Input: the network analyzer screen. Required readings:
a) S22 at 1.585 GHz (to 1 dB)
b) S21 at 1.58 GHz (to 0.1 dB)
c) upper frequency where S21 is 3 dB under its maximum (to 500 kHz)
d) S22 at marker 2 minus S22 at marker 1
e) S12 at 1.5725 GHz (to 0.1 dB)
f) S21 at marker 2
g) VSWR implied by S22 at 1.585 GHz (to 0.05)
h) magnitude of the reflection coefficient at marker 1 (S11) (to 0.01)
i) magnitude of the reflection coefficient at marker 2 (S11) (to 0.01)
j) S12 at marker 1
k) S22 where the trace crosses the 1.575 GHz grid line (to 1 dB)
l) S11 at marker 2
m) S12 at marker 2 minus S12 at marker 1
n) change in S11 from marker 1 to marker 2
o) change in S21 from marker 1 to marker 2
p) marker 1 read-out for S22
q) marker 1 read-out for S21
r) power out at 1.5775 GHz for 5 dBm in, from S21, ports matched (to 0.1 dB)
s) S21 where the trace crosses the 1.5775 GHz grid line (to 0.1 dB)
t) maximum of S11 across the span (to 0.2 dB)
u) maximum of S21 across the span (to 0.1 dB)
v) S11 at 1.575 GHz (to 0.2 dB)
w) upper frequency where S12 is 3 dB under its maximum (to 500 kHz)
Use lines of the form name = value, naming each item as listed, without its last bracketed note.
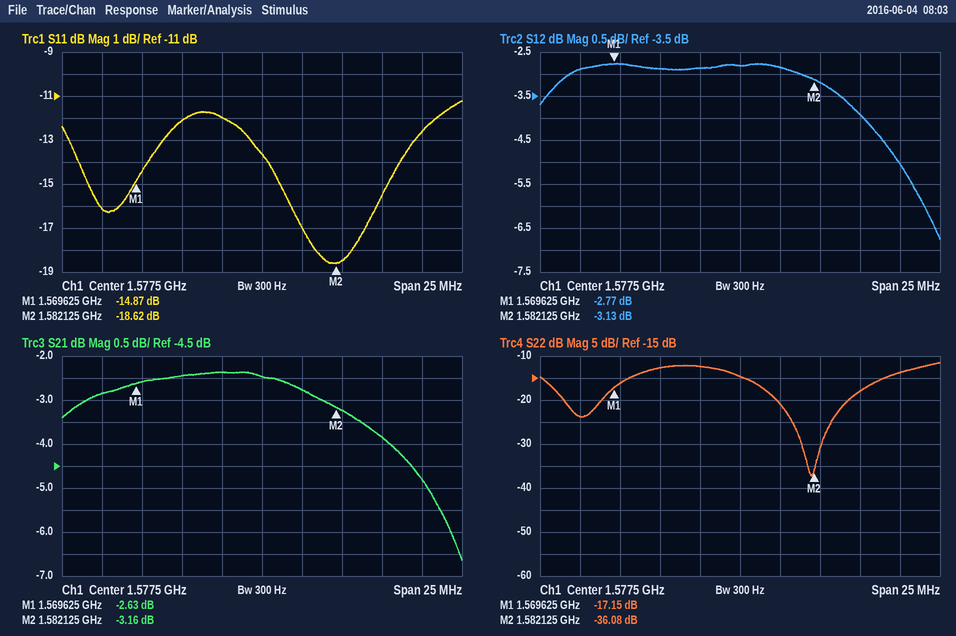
S22 at 1.585 GHz = -18 dB
S21 at 1.58 GHz = -2.8 dB
upper frequency where S21 is 3 dB under its maximum = 1.5885 GHz
S22 at marker 2 minus S22 at marker 1 = -18.93 dB
S12 at 1.5725 GHz = -2.9 dB
S21 at marker 2 = -3.16 dB
VSWR implied by S22 at 1.585 GHz = 1.30
magnitude of the reflection coefficient at marker 1 (S11) = 0.18
magnitude of the reflection coefficient at marker 2 (S11) = 0.12
S12 at marker 1 = -2.77 dB
S22 where the trace crosses the 1.575 GHz grid line = -12 dB
S11 at marker 2 = -18.62 dB
S12 at marker 2 minus S12 at marker 1 = -0.36 dB
change in S11 from marker 1 to marker 2 = -3.75 dB
change in S21 from marker 1 to marker 2 = -0.53 dB
marker 1 read-out for S22 = -17.15 dB
marker 1 read-out for S21 = -2.63 dB
power out at 1.5775 GHz for 5 dBm in, from S21, ports matched = 2.5 dBm
S21 where the trace crosses the 1.5775 GHz grid line = -2.5 dB
maximum of S11 across the span = -11.2 dB
maximum of S21 across the span = -2.4 dB
S11 at 1.575 GHz = -12.0 dB
upper frequency where S12 is 3 dB under its maximum = 1.5885 GHz
